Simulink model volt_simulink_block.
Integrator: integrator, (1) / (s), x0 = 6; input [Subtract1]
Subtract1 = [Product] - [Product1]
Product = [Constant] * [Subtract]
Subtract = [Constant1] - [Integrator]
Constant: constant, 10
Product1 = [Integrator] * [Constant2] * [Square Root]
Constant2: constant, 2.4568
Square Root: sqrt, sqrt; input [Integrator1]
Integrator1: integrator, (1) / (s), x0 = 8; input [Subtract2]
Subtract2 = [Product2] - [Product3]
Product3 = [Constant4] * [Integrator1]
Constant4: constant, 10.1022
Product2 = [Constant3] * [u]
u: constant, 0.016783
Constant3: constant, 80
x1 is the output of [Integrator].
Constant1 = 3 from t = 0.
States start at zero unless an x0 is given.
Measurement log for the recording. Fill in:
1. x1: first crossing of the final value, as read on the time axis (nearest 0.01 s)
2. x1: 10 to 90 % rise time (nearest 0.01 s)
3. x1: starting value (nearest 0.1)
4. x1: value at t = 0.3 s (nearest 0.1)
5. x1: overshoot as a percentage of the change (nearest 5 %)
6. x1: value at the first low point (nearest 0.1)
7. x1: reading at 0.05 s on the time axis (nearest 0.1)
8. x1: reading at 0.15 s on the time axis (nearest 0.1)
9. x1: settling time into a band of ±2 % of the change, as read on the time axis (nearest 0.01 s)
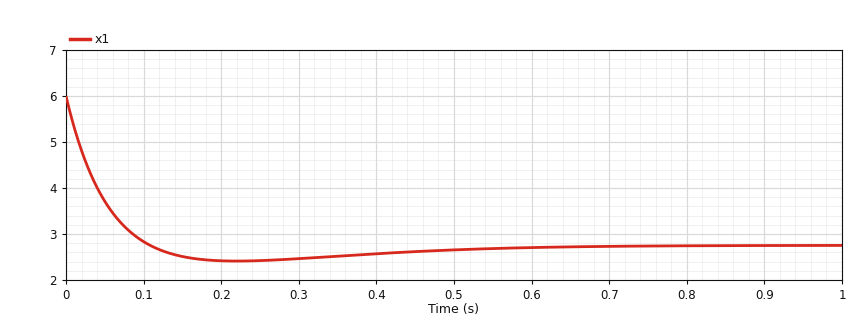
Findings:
0.11 s
0.08 s
6.0
2.5
10 %
2.4
3.7
2.5
0.56 s
